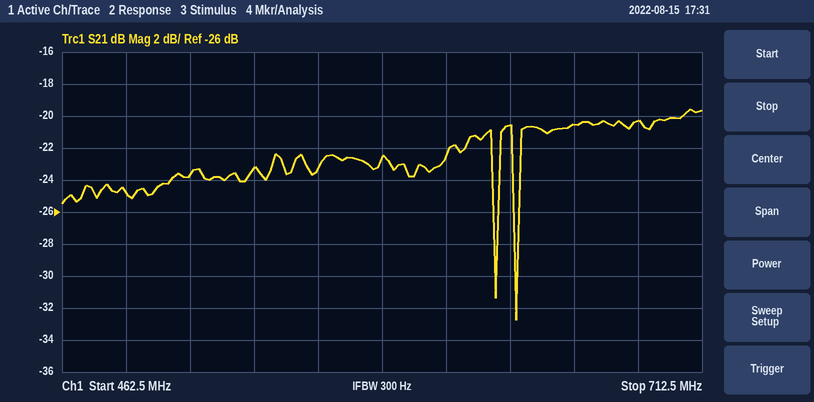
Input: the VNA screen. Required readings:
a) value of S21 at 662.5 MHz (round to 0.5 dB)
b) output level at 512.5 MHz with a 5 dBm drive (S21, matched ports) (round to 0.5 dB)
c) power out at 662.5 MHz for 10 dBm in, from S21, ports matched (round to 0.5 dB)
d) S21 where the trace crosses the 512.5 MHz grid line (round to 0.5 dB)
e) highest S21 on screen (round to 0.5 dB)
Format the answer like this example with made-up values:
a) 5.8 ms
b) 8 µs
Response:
a) -20.5 dB
b) -18.5 dBm
c) -10.5 dBm
d) -23.5 dB
e) -19.5 dB
